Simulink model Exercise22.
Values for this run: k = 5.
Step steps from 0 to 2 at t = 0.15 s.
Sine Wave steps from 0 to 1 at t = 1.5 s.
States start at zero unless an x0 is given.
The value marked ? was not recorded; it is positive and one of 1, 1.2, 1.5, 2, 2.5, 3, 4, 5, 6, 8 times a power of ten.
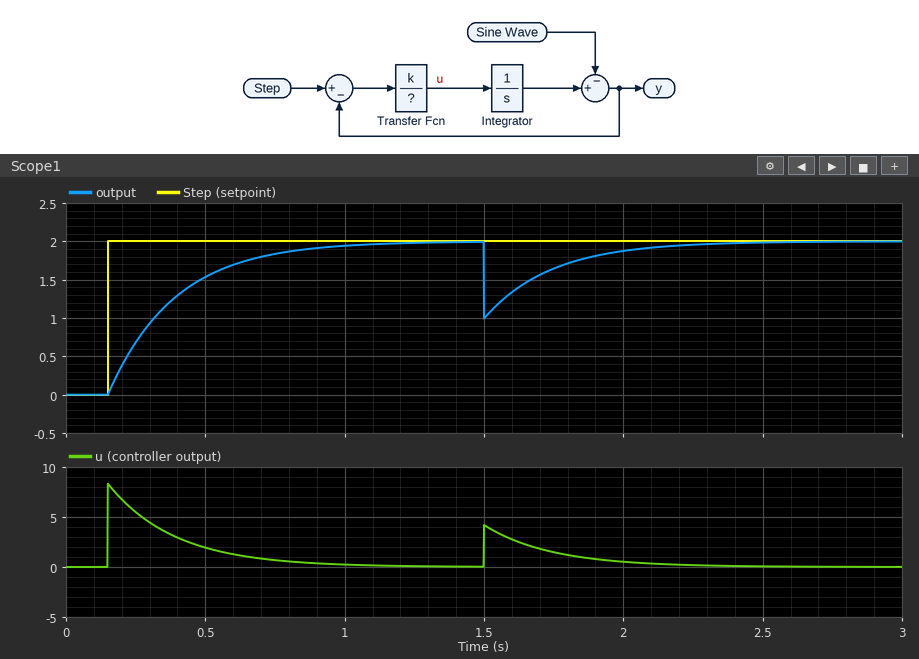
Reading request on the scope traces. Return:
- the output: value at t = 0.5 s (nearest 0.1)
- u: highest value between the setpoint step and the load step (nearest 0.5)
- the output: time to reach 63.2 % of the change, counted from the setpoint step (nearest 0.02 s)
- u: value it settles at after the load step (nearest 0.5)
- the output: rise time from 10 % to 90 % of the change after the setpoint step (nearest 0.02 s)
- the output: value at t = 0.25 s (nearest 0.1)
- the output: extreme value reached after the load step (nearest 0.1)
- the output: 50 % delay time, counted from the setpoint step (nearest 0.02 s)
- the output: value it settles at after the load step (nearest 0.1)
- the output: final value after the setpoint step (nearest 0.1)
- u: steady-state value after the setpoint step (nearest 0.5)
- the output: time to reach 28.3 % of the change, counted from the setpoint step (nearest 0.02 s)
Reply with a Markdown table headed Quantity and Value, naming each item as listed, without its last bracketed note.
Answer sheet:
| Quantity | Value |
|---|---|
| the output: value at t = 0.5 s | 1.5 |
| u: highest value between the setpoint step and the load step | 8.5 |
| the output: time to reach 63.2 % of the change, counted from the setpoint step | 0.24 s |
| u: value it settles at after the load step | 0.0 |
| the output: rise time from 10 % to 90 % of the change after the setpoint step | 0.52 s |
| the output: value at t = 0.25 s | 0.7 |
| the output: extreme value reached after the load step | 1.0 |
| the output: 50 % delay time, counted from the setpoint step | 0.16 s |
| the output: value it settles at after the load step | 2.0 |
| the output: final value after the setpoint step | 2.0 |
| u: steady-state value after the setpoint step | 0.0 |
| the output: time to reach 28.3 % of the change, counted from the setpoint step | 0.08 s |
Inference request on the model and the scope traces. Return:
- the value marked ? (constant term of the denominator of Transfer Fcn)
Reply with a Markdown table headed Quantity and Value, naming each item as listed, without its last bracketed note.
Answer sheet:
| Quantity | Value |
|---|---|
| the value marked ? | 1.2 |
